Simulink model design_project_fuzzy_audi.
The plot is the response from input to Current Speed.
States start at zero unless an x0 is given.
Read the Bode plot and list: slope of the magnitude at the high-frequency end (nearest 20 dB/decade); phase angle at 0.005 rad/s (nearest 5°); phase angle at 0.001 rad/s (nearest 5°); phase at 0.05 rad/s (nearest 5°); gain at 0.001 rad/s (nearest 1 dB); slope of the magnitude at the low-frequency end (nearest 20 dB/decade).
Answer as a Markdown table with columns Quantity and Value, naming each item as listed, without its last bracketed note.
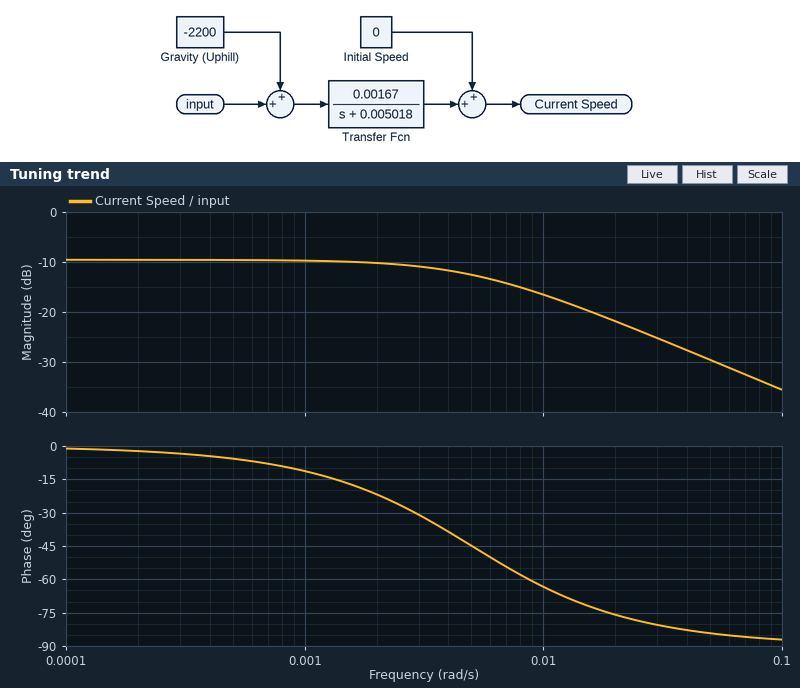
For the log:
| Quantity | Value |
|---|---|
| slope of the magnitude at the high-frequency end | -20 dB/decade |
| phase angle at 0.005 rad/s | -45° |
| phase angle at 0.001 rad/s | -10° |
| phase at 0.05 rad/s | -85° |
| gain at 0.001 rad/s | -10 dB |
| slope of the magnitude at the low-frequency end | 0 dB/decade |
